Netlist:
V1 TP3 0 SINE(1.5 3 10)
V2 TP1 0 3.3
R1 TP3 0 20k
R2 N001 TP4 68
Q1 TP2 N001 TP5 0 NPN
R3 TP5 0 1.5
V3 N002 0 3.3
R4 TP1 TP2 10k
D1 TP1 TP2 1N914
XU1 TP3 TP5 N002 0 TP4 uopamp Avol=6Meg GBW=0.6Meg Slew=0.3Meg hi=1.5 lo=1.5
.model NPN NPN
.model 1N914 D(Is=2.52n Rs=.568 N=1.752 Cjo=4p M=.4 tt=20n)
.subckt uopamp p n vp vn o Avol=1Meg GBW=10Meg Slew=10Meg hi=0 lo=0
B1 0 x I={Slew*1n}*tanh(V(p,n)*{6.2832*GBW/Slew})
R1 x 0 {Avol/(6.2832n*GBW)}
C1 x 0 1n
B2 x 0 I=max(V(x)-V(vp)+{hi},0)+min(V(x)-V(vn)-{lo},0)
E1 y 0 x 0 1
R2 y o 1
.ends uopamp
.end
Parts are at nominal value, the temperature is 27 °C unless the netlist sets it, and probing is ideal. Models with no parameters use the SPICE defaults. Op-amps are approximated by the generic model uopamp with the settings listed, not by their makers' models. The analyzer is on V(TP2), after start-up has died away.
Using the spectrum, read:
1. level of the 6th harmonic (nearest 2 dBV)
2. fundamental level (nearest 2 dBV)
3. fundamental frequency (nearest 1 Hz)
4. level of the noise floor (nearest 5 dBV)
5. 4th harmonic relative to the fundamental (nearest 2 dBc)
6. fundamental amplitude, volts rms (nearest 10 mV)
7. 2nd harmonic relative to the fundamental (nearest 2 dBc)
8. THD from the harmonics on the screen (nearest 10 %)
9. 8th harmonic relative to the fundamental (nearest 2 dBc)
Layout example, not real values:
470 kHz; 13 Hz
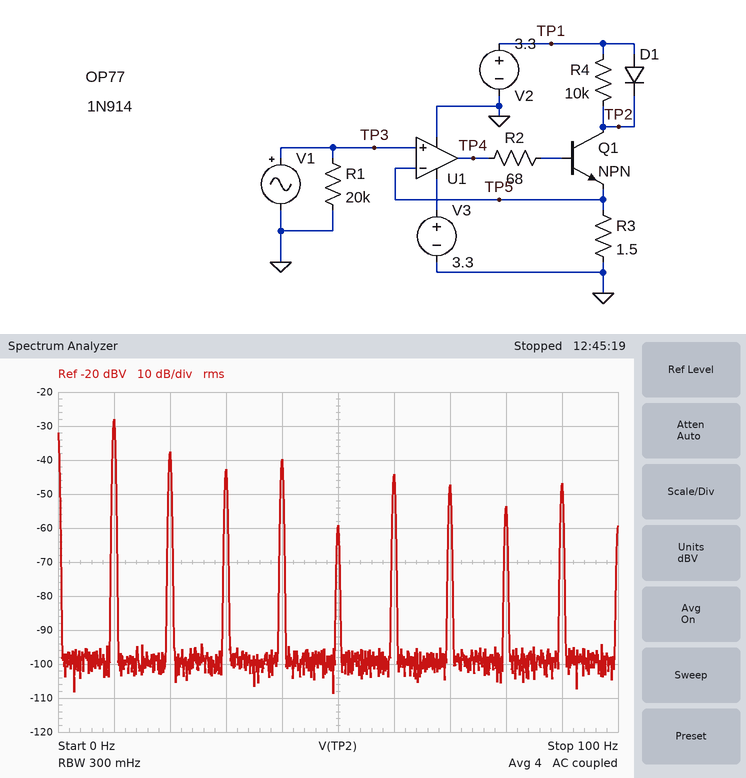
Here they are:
-44 dBV; -28 dBV; 10 Hz; -100 dBV; -12 dBc; 40 mV; -10 dBc; 50 %; -26 dBc
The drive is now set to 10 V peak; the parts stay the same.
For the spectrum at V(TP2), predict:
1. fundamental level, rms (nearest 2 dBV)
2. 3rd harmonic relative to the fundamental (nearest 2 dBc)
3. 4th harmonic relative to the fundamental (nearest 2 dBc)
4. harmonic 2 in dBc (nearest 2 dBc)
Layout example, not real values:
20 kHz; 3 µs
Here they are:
-28 dBV; -10 dBc; -20 dBc; -20 dBc
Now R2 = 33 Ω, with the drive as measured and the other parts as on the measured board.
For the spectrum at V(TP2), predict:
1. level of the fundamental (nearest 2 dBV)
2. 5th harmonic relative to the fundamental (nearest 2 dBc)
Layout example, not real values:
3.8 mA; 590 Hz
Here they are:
-26 dBV; -46 dBc
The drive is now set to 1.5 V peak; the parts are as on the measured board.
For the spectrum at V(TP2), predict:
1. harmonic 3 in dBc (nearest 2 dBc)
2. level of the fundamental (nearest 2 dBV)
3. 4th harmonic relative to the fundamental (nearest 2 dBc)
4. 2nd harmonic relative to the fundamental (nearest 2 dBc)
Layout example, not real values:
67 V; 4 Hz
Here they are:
-12 dBc; -30 dBV; -24 dBc; -4 dBc
